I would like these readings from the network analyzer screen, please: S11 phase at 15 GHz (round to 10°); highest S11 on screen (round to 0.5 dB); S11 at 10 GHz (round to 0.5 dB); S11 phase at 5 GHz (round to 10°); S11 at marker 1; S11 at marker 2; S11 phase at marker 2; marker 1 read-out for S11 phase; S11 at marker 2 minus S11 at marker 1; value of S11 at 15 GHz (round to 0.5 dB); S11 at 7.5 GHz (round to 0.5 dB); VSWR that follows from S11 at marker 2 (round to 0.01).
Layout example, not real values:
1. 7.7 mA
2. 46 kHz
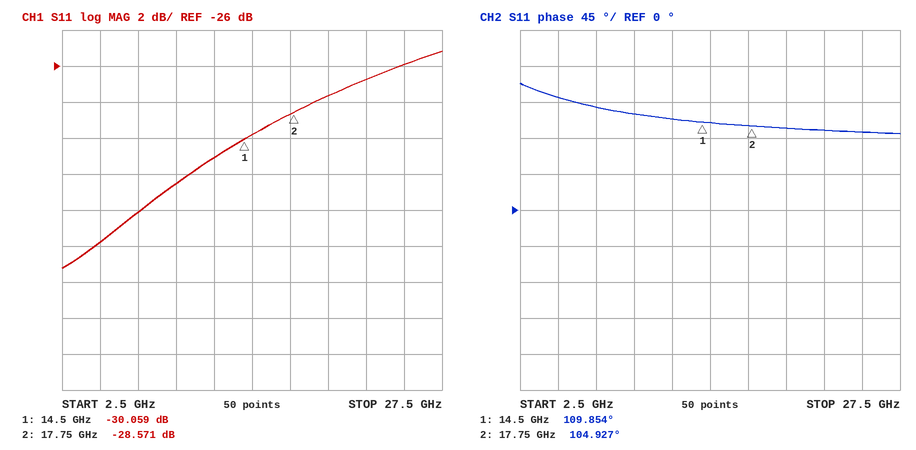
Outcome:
1. 110°
2. -25.0 dB
3. -32.5 dB
4. 140°
5. -30.059 dB
6. -28.571 dB
7. 104.927°
8. 109.854°
9. 1.488 dB
10. -30.0 dB
11. -34.0 dB
12. 1.08
